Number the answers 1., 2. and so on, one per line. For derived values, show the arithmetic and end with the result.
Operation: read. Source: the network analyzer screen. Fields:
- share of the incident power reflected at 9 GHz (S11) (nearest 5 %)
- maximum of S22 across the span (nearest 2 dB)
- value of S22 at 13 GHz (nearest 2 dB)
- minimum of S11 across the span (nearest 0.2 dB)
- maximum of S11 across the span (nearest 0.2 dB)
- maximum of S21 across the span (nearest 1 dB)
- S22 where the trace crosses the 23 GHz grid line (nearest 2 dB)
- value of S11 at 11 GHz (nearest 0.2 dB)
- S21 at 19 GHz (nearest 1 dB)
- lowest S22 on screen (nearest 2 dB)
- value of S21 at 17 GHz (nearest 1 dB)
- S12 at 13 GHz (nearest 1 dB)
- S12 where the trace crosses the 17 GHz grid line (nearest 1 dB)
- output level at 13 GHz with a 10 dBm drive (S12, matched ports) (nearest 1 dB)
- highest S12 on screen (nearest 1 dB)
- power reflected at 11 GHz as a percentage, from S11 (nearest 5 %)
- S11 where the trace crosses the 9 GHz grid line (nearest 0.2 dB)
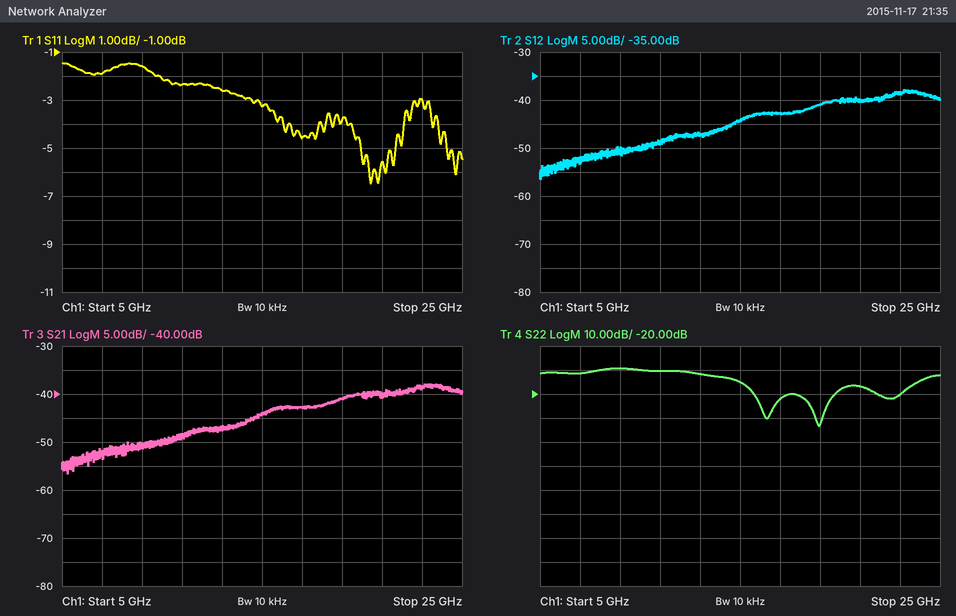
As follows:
1. 10^(-1.6/10) ≈ 69.2 %, so 70 % to the nearest 5 %
2. -10 dB
3. -12 dB
4. -6.4 dB
5. -1.4 dB
6. -38 dB
7. -20 dB
8. -2.4 dB
9. -41 dB
10. -34 dB
11. -43 dB
12. -47 dB
13. -43 dB
14. 10 dBm + (-47 dB) = -37 dBm
15. -38 dB
16. 10^(-2.4/10) ≈ 57.5 %, so 60 % to the nearest 5 %
17. -1.6 dB
